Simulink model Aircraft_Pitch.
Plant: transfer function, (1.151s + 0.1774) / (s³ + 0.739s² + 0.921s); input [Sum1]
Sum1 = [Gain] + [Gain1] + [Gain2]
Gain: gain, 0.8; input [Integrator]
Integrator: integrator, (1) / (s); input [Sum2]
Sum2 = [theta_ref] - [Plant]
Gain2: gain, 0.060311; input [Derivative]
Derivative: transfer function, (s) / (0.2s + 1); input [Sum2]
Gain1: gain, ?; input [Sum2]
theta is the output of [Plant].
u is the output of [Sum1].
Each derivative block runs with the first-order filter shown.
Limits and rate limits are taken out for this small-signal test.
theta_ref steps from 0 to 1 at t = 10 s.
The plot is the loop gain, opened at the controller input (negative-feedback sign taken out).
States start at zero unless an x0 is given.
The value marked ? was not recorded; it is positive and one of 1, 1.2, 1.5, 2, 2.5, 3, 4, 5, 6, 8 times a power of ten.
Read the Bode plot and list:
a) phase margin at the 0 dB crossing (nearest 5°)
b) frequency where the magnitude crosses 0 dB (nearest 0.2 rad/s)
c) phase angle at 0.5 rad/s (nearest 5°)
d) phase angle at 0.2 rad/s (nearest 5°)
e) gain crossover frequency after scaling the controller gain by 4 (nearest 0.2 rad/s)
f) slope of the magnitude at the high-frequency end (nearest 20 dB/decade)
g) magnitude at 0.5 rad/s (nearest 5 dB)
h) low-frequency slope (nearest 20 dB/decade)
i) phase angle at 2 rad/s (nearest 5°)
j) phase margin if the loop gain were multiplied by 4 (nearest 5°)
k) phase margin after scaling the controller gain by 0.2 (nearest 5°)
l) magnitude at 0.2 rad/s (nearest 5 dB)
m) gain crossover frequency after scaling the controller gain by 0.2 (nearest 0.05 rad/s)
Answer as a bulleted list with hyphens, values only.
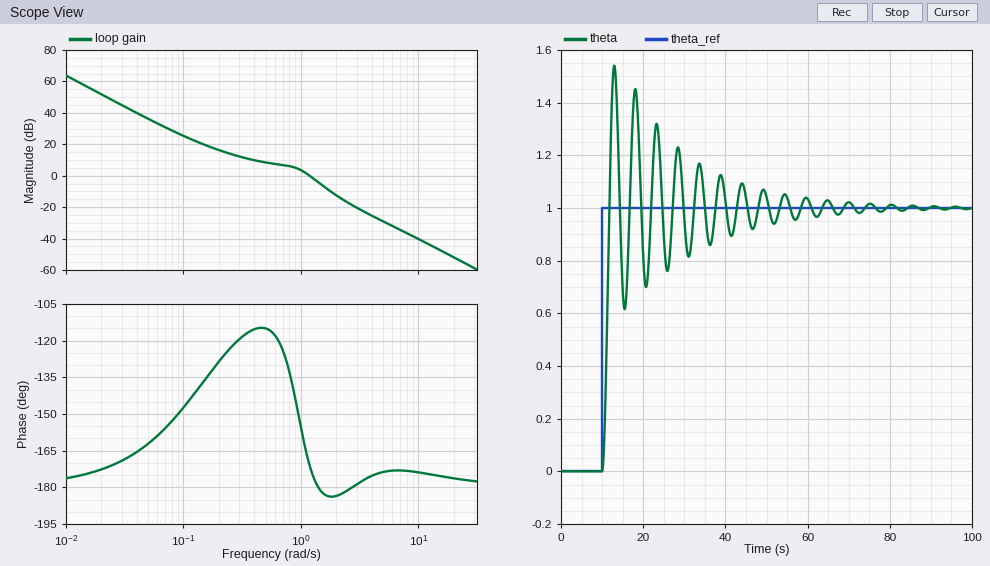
- 10°
- 1.2 rad/s
- -115°
- -130°
- 2.0 rad/s
- -40 dB/decade
- 10 dB
- -40 dB/decade
- -185°
- -5°
- 55°
- 15 dB
- 0.25 rad/s
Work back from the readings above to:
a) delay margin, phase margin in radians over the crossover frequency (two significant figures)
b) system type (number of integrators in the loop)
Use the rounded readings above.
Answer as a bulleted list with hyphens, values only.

- 0.15 s
- 2
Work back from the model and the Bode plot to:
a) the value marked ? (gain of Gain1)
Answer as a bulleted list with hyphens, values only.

- 0.6
